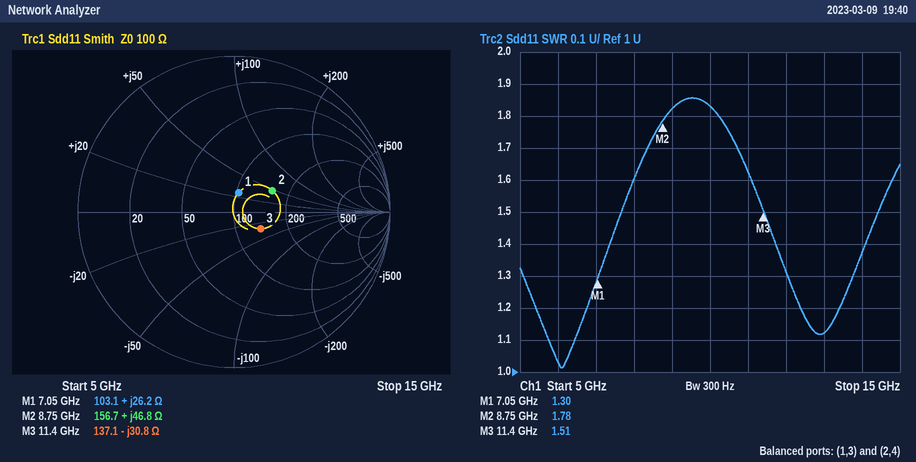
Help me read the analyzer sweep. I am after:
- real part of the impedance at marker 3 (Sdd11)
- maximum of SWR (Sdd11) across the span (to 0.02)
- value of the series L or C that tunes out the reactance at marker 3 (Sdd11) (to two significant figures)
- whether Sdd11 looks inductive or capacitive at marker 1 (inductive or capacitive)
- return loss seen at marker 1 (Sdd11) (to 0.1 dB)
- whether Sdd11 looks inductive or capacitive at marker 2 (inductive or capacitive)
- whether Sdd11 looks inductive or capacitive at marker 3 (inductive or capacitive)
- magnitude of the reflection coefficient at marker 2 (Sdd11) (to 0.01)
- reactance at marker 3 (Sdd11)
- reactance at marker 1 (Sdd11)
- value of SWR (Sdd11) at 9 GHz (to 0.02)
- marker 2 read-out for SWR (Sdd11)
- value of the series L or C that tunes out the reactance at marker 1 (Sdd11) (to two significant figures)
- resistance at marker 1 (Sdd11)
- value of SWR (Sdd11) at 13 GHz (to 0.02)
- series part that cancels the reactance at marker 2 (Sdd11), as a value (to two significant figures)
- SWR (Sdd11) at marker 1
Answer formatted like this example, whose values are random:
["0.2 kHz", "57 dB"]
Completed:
["137.1 Ω", "1.86", "430 pH", "inductive", "17.8 dB", "inductive", "capacitive", "0.28", "-30.8 Ω", "+26.2 Ω", "1.82", "1.78", "860 fF", "103.1 Ω", "1.12", "390 fF", "1.30"]
